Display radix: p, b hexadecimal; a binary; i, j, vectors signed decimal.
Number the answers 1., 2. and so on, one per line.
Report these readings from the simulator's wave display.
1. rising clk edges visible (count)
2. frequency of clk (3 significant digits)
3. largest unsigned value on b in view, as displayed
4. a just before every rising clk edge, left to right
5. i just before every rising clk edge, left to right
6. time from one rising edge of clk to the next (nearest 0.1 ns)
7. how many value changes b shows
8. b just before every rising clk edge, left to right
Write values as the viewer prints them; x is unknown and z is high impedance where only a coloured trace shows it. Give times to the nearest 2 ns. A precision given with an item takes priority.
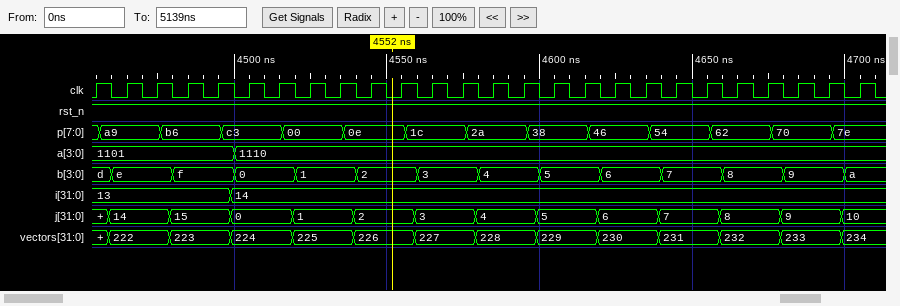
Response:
1. 26
2. 100 MHz
3. f
4. 1101, 1101, 1101, 1101, 1101, 1110, 1110, 1110, 1110, 1110, 1110, 1110, 1110, 1110, 1110, 1110, 1110, 1110, 1110, 1110, 1110, 1110, 1110, 1110, 1110, 1110
5. 13, 13, 13, 13, 13, 14, 14, 14, 14, 14, 14, 14, 14, 14, 14, 14, 14, 14, 14, 14, 14, 14, 14, 14, 14, 14
6. 10 ns
7. 13
8. d, e, e, f, f, 0, 0, 1, 1, 2, 2, 3, 3, 4, 4, 5, 5, 6, 6, 7, 7, 8, 8, 9, 9, a
